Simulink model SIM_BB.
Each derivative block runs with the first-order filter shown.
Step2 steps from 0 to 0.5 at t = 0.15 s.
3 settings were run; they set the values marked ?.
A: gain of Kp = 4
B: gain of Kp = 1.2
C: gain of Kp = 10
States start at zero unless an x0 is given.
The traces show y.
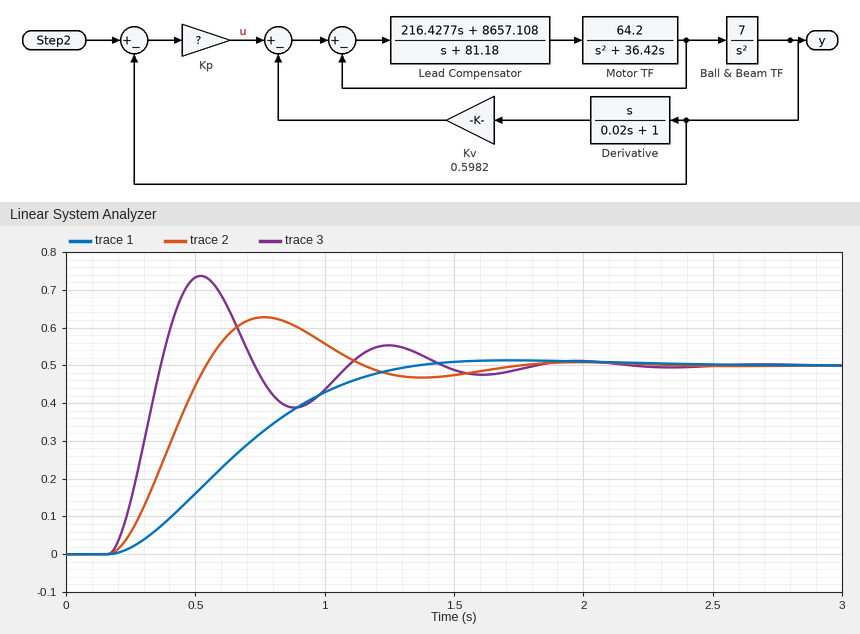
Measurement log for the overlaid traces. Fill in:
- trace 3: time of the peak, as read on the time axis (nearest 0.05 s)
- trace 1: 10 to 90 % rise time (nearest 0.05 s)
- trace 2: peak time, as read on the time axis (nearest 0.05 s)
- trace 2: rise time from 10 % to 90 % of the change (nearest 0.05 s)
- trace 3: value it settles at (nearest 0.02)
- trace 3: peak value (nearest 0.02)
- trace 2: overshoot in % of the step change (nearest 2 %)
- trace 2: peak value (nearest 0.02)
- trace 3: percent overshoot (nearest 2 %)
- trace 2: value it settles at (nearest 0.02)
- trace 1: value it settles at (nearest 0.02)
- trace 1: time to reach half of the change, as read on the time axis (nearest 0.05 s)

0.50 s
0.75 s
0.75 s
0.25 s
0.50
0.74
26 %
0.62
48 %
0.50
0.50
0.65 s
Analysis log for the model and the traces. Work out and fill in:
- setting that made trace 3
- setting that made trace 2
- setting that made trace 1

C
A
B
